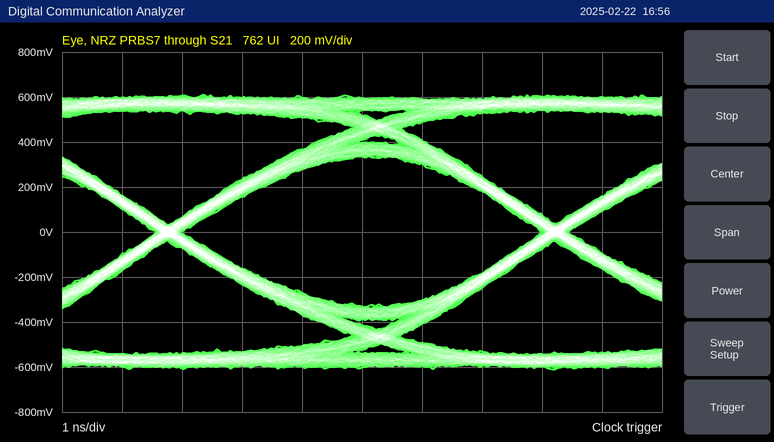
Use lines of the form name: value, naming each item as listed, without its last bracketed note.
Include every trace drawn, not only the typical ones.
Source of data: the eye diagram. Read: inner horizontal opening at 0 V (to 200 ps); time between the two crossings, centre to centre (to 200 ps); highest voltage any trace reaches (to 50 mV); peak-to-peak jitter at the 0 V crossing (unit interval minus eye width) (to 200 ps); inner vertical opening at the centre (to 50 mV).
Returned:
inner horizontal opening at 0 V: 6.0 ns
time between the two crossings, centre to centre: 6.4 ns
highest voltage any trace reaches: 600 mV
peak-to-peak jitter at the 0 V crossing (unit interval minus eye width): 400 ps
inner vertical opening at the centre: 650 mV
